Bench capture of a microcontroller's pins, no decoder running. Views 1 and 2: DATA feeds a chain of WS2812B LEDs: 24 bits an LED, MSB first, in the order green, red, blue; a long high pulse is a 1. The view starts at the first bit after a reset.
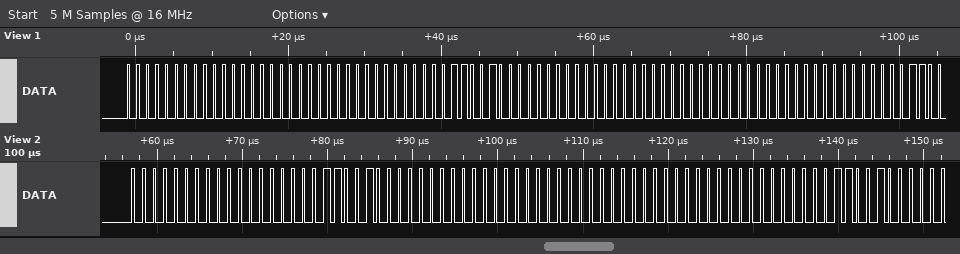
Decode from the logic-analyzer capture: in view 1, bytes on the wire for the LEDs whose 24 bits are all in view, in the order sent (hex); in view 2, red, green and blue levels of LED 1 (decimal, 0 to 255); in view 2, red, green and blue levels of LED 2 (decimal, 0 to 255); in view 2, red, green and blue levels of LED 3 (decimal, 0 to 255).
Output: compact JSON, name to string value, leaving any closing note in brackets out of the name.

{"in view 1, bytes on the wire for the LEDs whose 24 bits are all in view, in the order sent": "00 00 00 00 32 00 00 00 00", "in view 2, red, green and blue levels of LED 1": "0, 0, 50", "in view 2, red, green and blue levels of LED 2": "0, 0, 0", "in view 2, red, green and blue levels of LED 3": "0, 0, 50"}
